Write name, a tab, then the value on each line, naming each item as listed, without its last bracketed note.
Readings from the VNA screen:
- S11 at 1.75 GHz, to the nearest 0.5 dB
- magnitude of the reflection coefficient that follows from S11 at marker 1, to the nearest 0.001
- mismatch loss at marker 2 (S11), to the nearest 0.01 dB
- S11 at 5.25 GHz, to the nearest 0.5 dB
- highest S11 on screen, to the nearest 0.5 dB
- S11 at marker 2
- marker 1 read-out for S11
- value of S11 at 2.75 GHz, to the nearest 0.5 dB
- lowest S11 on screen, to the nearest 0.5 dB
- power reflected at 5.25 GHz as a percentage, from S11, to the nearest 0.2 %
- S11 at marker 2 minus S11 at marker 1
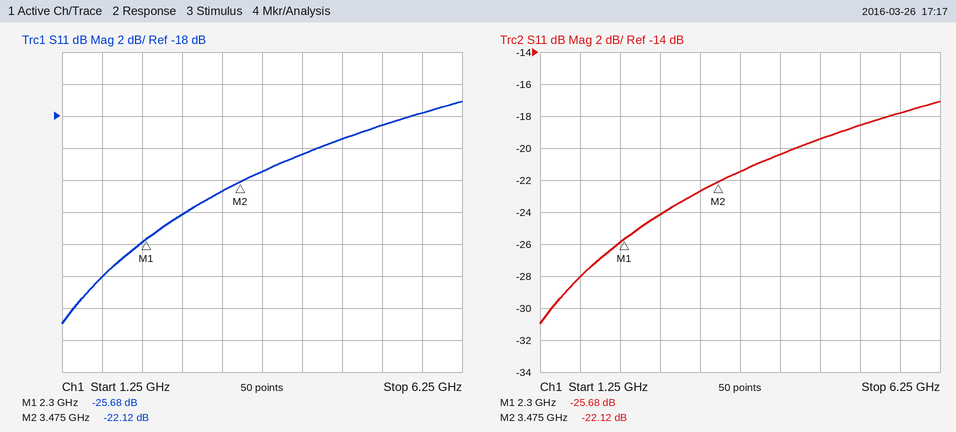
S11 at 1.75 GHz, to the nearest 0.5 dB	-28.0 dB
magnitude of the reflection coefficient that follows from S11 at marker 1, to the nearest 0.001	0.052
mismatch loss at marker 2 (S11), to the nearest 0.01 dB	0.03 dB
S11 at 5.25 GHz, to the nearest 0.5 dB	-18.5 dB
highest S11 on screen, to the nearest 0.5 dB	-17.0 dB
S11 at marker 2	-22.12 dB
marker 1 read-out for S11	-25.68 dB
value of S11 at 2.75 GHz, to the nearest 0.5 dB	-24.0 dB
lowest S11 on screen, to the nearest 0.5 dB	-31.0 dB
power reflected at 5.25 GHz as a percentage, from S11, to the nearest 0.2 %	1.4 %
S11 at marker 2 minus S11 at marker 1	3.56 dB
